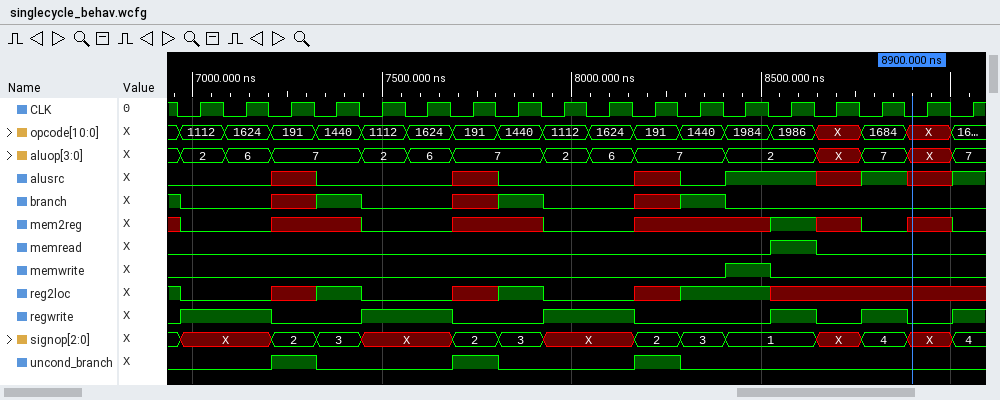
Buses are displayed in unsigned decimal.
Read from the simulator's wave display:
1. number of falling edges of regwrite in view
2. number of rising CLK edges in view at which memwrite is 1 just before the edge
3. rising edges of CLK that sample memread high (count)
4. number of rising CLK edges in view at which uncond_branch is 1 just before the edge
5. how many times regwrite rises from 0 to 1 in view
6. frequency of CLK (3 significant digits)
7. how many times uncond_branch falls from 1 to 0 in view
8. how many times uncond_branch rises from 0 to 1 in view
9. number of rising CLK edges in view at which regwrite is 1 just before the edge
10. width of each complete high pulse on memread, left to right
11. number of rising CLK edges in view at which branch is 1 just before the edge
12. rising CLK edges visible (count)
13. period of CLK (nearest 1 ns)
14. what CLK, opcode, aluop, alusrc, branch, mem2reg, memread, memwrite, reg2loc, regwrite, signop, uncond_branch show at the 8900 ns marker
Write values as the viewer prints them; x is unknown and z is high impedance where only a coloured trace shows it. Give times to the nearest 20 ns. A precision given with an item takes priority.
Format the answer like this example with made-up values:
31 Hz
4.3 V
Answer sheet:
5
1
1
3
6
8.33 MHz
3
3
9
120 ns
3
18
120 ns
CLK=0, opcode=X, aluop=X, alusrc=x, branch=0, mem2reg=x, memread=0, memwrite=0, reg2loc=x, regwrite=0, signop=X, uncond_branch=0
